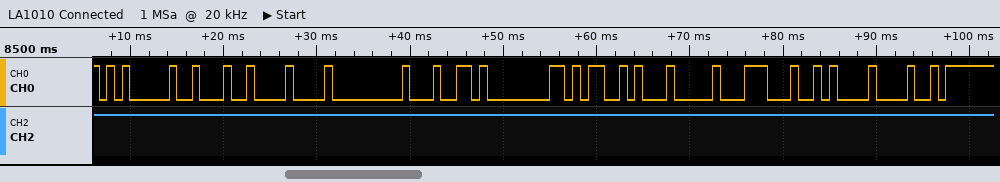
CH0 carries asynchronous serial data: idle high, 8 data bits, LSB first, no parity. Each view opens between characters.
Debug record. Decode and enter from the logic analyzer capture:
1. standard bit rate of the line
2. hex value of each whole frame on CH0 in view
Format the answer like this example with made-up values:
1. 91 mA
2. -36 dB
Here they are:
1. 1200 baud
2. 05, 22, 08, 00, 64, 80, 4D, 04, 1C, 0A, 48
